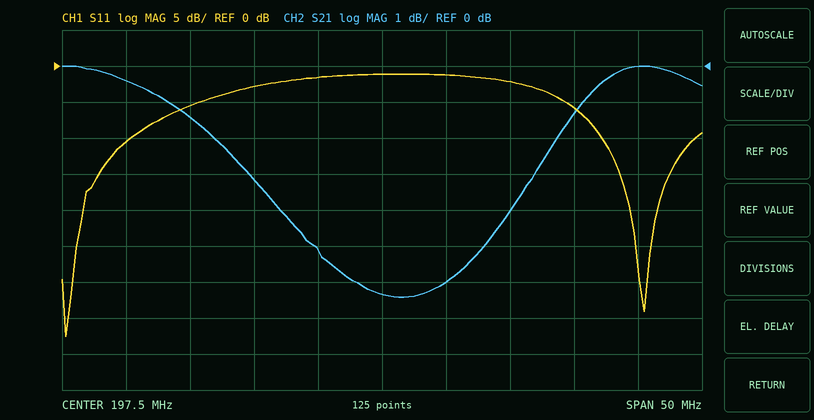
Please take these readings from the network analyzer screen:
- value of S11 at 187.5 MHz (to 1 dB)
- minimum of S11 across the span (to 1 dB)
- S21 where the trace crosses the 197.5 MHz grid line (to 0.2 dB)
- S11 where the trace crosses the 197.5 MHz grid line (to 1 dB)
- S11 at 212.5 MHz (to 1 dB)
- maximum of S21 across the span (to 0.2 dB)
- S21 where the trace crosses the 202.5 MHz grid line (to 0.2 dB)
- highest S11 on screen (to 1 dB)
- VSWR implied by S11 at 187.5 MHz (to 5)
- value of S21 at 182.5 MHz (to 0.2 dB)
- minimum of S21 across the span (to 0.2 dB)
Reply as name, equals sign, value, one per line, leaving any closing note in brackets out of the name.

value of S11 at 187.5 MHz = -3 dB
minimum of S11 across the span = -38 dB
S21 where the trace crosses the 197.5 MHz grid line = -6.4 dB
S11 where the trace crosses the 197.5 MHz grid line = -1 dB
S11 at 212.5 MHz = -6 dB
maximum of S21 across the span = 0.0 dB
S21 where the trace crosses the 202.5 MHz grid line = -6.0 dB
highest S11 on screen = -1 dB
VSWR implied by S11 at 187.5 MHz = 5
value of S21 at 182.5 MHz = -1.4 dB
minimum of S21 across the span = -6.4 dB
